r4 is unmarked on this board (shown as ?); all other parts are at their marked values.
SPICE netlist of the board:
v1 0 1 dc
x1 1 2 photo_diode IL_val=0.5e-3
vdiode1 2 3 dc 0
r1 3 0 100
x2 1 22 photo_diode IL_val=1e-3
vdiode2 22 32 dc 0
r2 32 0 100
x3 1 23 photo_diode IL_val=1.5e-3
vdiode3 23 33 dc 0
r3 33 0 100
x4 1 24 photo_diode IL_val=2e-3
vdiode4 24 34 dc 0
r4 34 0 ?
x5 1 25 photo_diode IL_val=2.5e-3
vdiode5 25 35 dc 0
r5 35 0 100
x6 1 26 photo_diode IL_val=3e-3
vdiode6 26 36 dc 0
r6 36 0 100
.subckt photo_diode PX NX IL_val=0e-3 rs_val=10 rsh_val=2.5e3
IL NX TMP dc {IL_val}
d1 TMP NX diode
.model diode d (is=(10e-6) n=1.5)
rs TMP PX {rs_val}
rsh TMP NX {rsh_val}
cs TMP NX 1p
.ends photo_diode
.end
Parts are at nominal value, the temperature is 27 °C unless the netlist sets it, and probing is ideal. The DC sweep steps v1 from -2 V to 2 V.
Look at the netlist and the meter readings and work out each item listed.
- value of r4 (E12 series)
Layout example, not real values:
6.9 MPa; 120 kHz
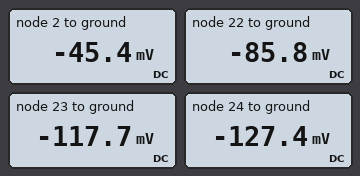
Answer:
82 Ω
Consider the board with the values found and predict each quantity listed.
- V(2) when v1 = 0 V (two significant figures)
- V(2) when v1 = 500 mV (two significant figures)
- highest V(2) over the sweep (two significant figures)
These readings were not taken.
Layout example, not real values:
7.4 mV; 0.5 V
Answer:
-45 mV; -68 mV; 1.6 V
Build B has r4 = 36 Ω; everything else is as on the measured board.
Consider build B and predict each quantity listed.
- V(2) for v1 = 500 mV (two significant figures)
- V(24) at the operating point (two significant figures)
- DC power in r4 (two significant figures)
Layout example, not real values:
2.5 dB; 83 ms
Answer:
-68 mV; -68 mV; 130 µW
